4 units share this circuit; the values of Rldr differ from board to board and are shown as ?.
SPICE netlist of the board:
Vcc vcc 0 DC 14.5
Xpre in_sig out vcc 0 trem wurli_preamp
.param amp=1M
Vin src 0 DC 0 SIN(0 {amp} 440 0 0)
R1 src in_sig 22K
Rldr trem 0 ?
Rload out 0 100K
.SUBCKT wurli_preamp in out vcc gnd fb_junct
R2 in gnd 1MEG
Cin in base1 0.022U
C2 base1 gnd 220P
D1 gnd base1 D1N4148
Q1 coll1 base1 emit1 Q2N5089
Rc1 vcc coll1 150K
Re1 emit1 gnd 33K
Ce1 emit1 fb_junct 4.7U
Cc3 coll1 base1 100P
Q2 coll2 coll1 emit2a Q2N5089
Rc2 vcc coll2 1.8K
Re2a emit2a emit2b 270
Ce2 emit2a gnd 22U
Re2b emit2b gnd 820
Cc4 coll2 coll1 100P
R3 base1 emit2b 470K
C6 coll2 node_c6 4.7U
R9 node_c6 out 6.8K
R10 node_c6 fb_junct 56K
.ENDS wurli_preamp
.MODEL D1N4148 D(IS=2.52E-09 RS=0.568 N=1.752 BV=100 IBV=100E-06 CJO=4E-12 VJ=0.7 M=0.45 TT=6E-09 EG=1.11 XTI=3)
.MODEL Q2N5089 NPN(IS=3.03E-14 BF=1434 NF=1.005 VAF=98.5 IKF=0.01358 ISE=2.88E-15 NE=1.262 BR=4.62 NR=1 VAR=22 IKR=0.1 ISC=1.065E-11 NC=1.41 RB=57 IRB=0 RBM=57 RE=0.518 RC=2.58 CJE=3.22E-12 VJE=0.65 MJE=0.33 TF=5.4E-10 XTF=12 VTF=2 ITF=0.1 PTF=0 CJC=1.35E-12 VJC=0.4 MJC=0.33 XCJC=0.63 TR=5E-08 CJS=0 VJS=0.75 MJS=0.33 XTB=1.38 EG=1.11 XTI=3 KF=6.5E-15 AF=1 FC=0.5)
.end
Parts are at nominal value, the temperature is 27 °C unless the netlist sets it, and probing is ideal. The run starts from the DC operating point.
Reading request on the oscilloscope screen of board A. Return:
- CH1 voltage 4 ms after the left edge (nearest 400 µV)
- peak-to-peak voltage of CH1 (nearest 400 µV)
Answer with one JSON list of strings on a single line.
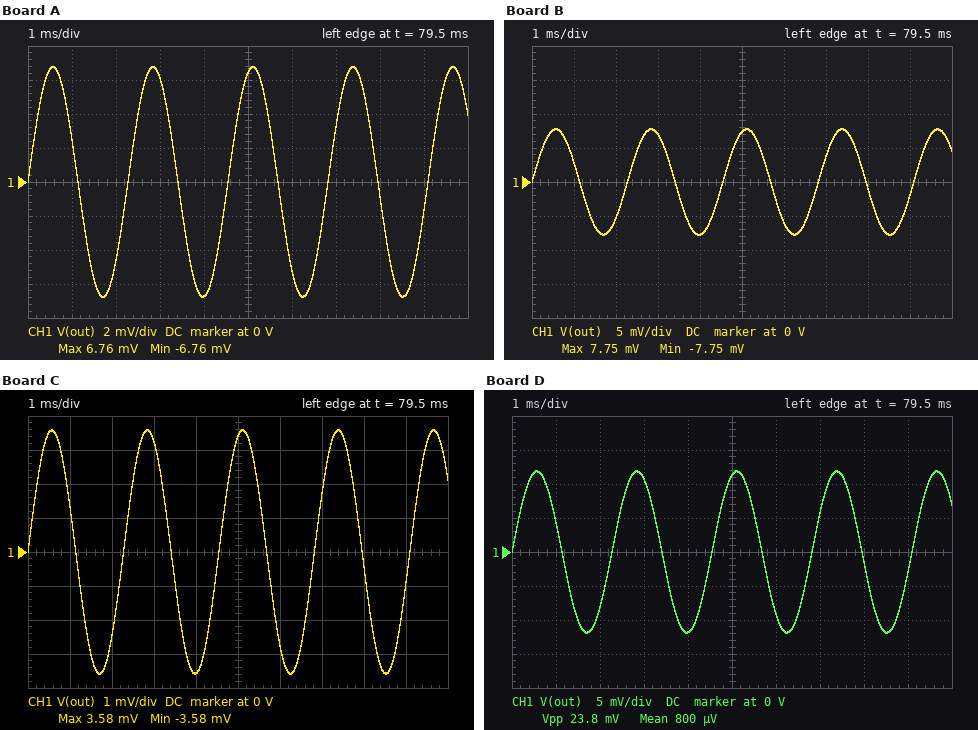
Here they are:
["-6.8 mV", "13.6 mV"]
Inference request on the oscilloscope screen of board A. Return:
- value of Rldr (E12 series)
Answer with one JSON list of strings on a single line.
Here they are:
["10 kΩ"]
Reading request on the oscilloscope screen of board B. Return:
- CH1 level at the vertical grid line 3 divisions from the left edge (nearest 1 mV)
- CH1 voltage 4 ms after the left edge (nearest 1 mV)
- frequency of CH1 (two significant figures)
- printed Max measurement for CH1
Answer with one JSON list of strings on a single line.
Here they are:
["7 mV", "-8 mV", "440 Hz", "7.75 mV"]
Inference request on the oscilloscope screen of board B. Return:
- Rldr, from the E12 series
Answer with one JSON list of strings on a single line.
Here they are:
["8.2 kΩ"]
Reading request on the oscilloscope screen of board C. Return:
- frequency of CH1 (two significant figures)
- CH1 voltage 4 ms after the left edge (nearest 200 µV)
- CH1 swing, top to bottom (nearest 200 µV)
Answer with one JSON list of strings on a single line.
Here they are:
["440 Hz", "-3.6 mV", "7.2 mV"]
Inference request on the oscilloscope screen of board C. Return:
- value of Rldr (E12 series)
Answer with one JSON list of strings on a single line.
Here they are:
["33 kΩ"]
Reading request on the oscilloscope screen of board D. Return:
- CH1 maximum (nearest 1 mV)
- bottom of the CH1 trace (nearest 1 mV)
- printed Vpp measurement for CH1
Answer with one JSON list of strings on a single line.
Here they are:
["12 mV", "-12 mV", "23.8 mV"]
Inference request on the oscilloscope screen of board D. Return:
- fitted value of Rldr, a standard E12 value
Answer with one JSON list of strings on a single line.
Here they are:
["4.7 kΩ"]
